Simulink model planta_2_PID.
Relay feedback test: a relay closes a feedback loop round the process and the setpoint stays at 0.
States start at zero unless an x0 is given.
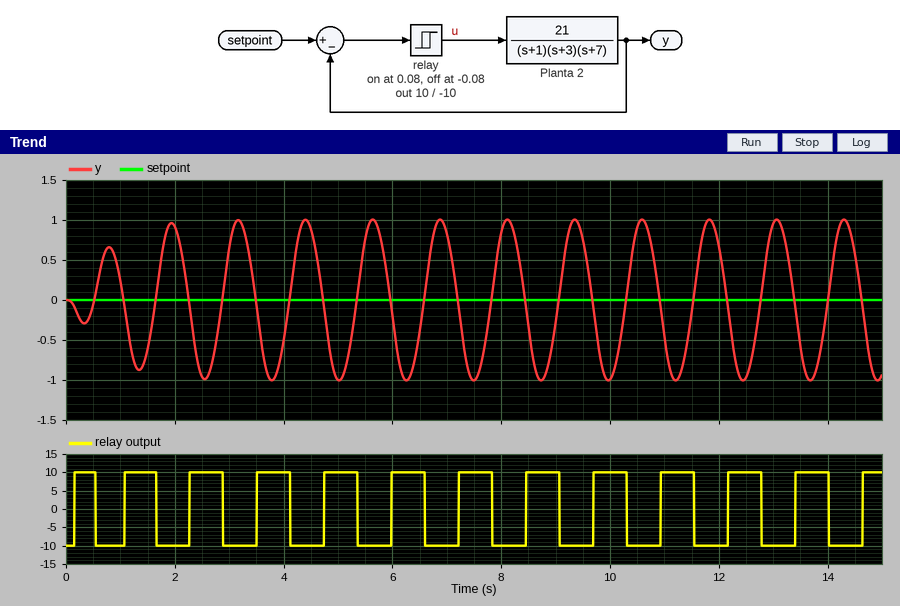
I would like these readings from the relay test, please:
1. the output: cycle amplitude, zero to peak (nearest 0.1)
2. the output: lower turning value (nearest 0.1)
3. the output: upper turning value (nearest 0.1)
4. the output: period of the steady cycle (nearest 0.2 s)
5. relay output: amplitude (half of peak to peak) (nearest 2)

1.0
-1.0
1.0
1.2 s
10
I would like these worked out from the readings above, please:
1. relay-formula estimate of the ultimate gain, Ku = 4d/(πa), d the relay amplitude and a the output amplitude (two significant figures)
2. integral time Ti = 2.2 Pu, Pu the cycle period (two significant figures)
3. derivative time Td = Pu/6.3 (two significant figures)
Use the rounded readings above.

13
2.6 s
0.19 s
